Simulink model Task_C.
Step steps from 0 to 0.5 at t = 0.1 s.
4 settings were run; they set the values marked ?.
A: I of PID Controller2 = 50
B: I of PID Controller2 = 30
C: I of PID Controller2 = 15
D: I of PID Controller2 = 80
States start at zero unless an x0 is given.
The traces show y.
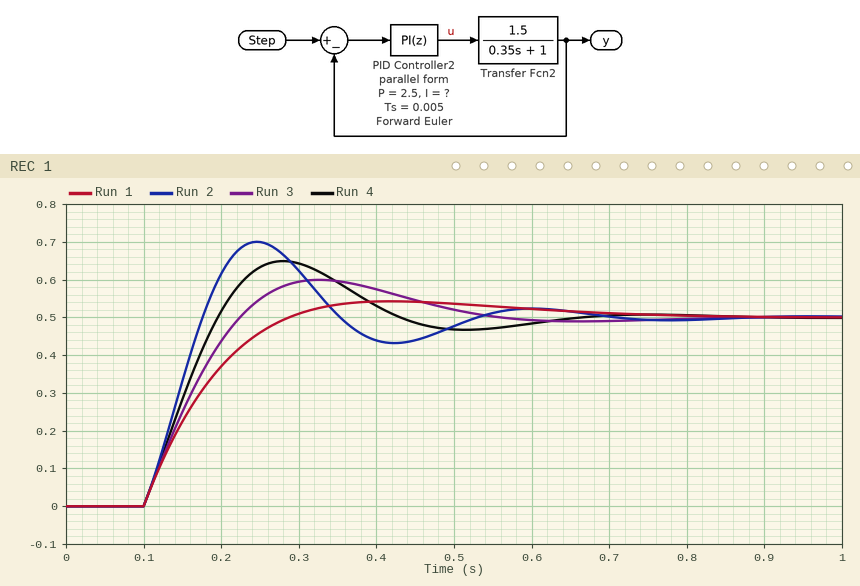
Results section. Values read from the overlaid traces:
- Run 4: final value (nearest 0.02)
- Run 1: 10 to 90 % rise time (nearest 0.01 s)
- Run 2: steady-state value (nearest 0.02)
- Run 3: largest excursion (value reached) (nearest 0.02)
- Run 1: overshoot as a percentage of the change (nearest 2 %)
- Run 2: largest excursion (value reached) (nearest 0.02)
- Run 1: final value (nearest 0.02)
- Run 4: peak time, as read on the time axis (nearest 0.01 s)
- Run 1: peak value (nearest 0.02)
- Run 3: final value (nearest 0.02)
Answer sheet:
0.50
0.13 s
0.50
0.60
8 %
0.70
0.50
0.28 s
0.54
0.50
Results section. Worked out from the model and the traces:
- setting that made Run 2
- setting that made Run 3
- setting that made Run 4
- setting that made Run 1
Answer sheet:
D
B
A
C
